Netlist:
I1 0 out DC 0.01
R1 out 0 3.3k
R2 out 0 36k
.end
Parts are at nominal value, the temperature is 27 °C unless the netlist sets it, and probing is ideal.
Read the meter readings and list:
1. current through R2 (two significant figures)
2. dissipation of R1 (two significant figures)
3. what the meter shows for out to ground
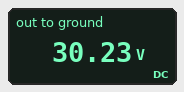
840 µA
280 mW
30.23 V
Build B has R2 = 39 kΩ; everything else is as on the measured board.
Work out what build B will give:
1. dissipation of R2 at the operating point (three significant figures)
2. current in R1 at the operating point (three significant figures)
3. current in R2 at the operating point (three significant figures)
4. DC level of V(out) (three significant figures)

23.7 mW
9.22 mA
780 µA
30.4 V
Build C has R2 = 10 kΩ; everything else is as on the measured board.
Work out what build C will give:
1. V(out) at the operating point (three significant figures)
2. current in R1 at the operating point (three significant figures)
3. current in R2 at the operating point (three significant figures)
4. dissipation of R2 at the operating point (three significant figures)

24.8 V
7.52 mA
2.48 mA
61.6 mW
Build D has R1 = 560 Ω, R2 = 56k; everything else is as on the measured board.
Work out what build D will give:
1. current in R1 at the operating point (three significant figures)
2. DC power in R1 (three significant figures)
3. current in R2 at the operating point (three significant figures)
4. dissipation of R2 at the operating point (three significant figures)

9.90 mA
54.9 mW
99.0 µA
549 µW
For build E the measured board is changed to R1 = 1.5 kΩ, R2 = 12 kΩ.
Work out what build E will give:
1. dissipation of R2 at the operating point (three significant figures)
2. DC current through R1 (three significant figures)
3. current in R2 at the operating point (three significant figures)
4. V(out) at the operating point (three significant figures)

14.8 mW
8.89 mA
1.11 mA
13.3 V
